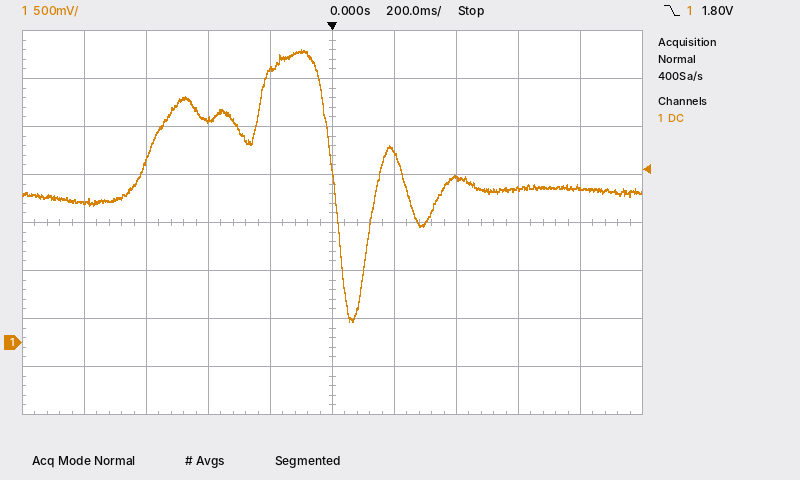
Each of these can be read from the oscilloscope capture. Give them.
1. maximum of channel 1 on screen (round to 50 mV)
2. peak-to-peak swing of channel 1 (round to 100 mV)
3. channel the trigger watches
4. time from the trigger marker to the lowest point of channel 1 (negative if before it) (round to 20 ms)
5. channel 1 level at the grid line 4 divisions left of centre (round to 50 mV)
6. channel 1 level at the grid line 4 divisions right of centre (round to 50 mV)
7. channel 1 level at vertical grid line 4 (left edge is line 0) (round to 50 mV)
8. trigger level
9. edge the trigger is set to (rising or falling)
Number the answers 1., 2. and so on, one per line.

1. 3.05 V
2. 2.80 V
3. channel 1
4. +60 ms
5. 1.45 V
6. 1.60 V
7. 2.85 V
8. 1.80 V
9. falling
